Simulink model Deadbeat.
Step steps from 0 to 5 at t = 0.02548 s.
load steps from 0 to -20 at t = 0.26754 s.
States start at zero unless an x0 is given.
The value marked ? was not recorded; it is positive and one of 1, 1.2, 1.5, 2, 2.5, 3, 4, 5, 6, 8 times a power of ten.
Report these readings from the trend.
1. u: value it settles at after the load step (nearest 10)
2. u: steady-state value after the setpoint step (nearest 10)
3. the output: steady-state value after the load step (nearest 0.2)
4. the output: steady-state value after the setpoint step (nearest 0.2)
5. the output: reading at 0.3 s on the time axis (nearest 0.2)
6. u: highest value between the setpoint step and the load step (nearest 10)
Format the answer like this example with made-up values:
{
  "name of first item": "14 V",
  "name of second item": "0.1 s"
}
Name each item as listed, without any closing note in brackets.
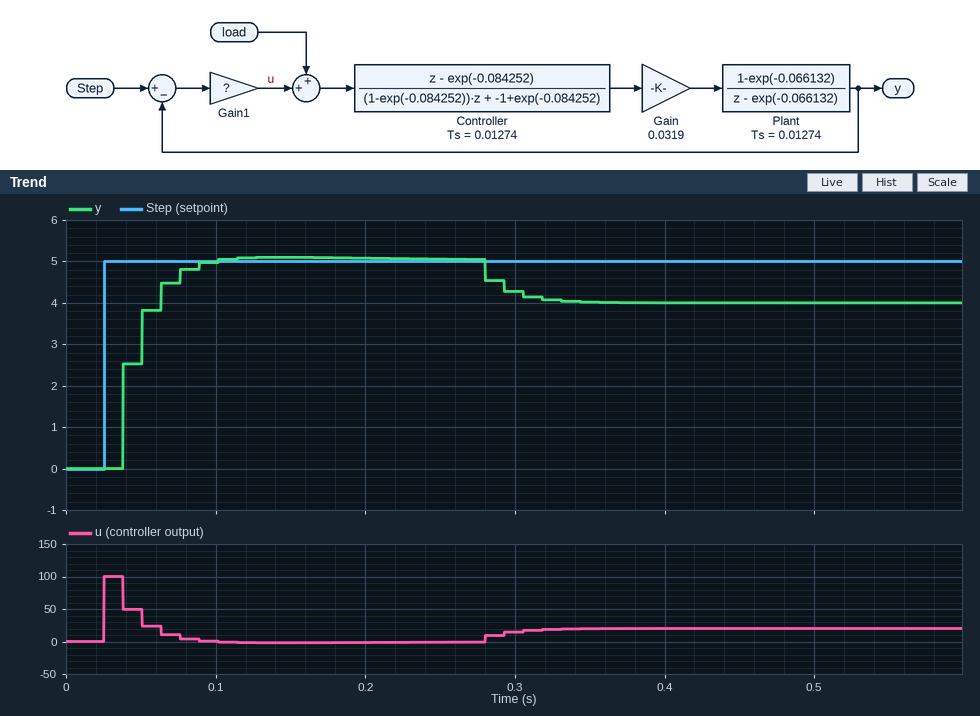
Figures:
{
  "u: value it settles at after the load step": "20",
  "u: steady-state value after the setpoint step": "0",
  "the output: steady-state value after the load step": "4.0",
  "the output: steady-state value after the setpoint step": "5.0",
  "the output: reading at 0.3 s on the time axis": "4.2",
  "u: highest value between the setpoint step and the load step": "100"
}
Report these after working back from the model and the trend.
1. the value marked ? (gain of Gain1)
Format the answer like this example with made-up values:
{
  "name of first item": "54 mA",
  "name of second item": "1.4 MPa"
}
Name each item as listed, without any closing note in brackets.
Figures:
{
  "the value marked ?": "20"
}
